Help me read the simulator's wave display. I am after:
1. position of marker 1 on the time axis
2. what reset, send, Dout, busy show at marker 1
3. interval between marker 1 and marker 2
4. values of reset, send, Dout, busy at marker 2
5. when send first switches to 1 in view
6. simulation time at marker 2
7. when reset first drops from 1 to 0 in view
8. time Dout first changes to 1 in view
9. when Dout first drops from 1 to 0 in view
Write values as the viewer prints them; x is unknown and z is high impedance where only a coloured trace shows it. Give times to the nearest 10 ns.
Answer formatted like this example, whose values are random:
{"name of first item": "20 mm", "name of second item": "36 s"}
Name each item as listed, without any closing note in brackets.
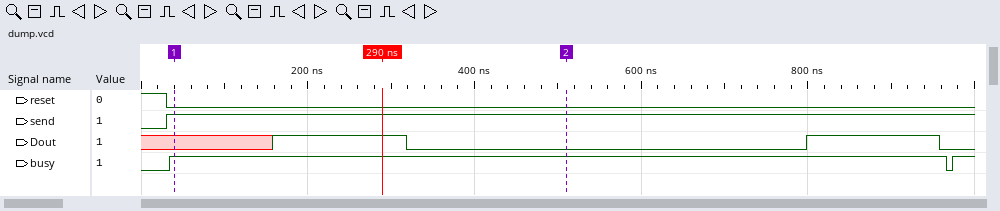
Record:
{"position of marker 1 on the time axis": "40 ns", "what reset, send, Dout, busy show at marker 1": "reset=0, send=1, Dout=x, busy=1", "interval between marker 1 and marker 2": "470 ns", "values of reset, send, Dout, busy at marker 2": "reset=0, send=1, Dout=0, busy=1", "when send first switches to 1 in view": "30 ns", "simulation time at marker 2": "510 ns", "when reset first drops from 1 to 0 in view": "30 ns", "time Dout first changes to 1 in view": "160 ns", "when Dout first drops from 1 to 0 in view": "320 ns"}
